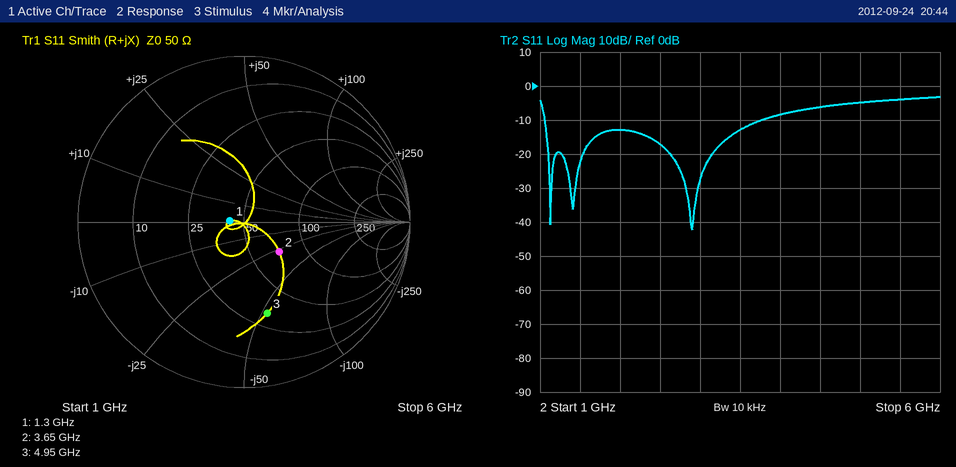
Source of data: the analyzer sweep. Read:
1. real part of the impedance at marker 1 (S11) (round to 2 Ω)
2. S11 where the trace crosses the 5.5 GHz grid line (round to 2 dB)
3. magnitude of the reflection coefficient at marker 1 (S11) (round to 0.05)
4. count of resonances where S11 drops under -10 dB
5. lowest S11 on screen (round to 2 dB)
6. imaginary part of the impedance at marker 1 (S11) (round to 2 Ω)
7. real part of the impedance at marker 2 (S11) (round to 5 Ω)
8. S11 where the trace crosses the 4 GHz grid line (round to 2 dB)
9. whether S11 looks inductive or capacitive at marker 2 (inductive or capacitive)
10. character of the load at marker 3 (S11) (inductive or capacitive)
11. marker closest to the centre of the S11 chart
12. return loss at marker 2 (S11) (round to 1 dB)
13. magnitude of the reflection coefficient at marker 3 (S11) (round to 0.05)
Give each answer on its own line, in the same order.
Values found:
42 Ω
-4 dB
0.10
3
-42 dB
0 Ω
70 Ω
-8 dB
capacitive
capacitive
marker 1
11 dB
0.55
